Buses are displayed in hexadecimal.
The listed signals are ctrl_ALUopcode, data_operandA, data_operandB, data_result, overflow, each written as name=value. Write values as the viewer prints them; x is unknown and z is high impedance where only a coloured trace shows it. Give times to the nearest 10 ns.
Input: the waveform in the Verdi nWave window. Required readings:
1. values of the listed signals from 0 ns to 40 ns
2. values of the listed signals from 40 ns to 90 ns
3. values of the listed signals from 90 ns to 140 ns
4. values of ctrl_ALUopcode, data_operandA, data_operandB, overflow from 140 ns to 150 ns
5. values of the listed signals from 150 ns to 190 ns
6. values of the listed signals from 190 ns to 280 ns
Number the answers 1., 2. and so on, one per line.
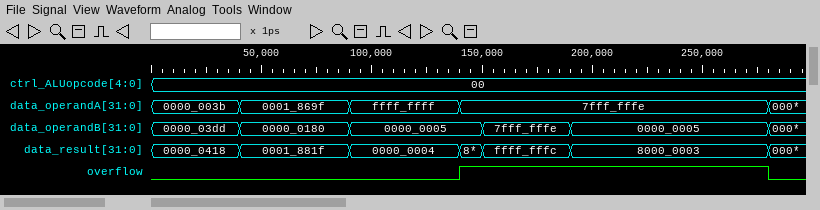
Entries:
1. ctrl_ALUopcode=00, data_operandA=0000_003b, data_operandB=0000_03dd, data_result=0000_0418, overflow=0
2. ctrl_ALUopcode=00, data_operandA=0001_869f, data_operandB=0000_0180, data_result=0001_881f, overflow=0
3. ctrl_ALUopcode=00, data_operandA=ffff_ffff, data_operandB=0000_0005, data_result=0000_0004, overflow=0
4. ctrl_ALUopcode=00, data_operandA=7fff_fffe, data_operandB=0000_0005, overflow=1
5. ctrl_ALUopcode=00, data_operandA=7fff_fffe, data_operandB=7fff_fffe, data_result=ffff_fffc, overflow=1
6. ctrl_ALUopcode=00, data_operandA=7fff_fffe, data_operandB=0000_0005, data_result=8000_0003, overflow=1
